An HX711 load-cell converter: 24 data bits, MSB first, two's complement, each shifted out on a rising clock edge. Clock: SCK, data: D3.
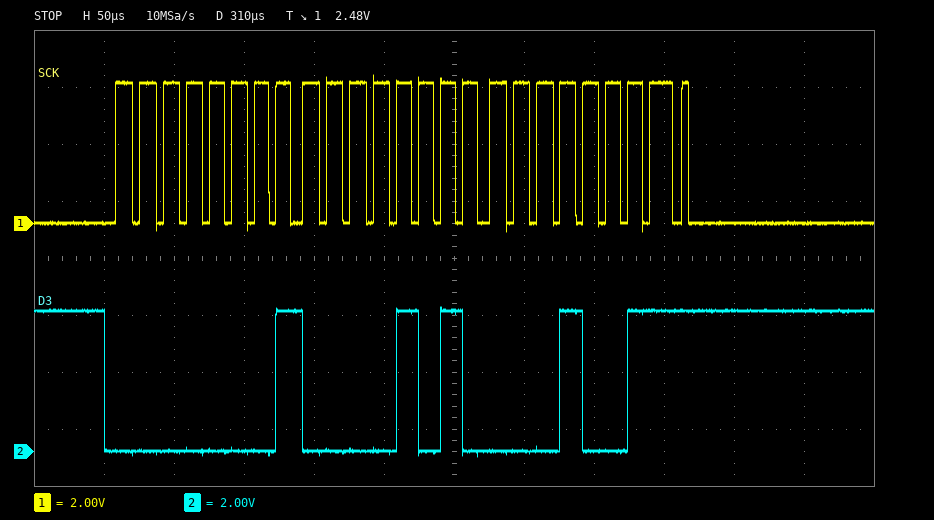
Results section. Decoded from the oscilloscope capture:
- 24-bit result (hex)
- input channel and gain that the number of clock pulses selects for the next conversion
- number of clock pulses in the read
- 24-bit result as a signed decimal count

0x010A13
channel A, gain 128
25
68115
